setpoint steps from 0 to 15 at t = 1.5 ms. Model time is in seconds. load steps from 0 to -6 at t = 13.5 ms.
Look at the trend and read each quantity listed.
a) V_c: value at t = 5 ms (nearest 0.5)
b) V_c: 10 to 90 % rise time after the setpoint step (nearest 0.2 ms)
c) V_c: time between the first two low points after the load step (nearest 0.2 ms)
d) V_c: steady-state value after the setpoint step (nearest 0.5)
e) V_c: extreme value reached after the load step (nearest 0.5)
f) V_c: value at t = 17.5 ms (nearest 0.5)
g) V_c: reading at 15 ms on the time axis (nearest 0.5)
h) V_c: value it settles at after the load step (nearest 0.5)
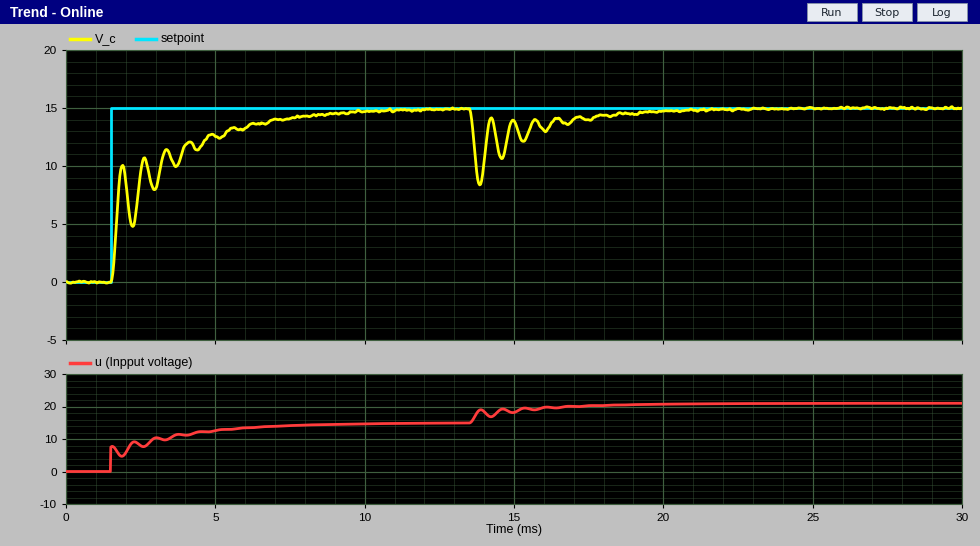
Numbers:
12.5
4.6 ms
0.8 ms
15.0
8.5
14.0
14.0
15.0
